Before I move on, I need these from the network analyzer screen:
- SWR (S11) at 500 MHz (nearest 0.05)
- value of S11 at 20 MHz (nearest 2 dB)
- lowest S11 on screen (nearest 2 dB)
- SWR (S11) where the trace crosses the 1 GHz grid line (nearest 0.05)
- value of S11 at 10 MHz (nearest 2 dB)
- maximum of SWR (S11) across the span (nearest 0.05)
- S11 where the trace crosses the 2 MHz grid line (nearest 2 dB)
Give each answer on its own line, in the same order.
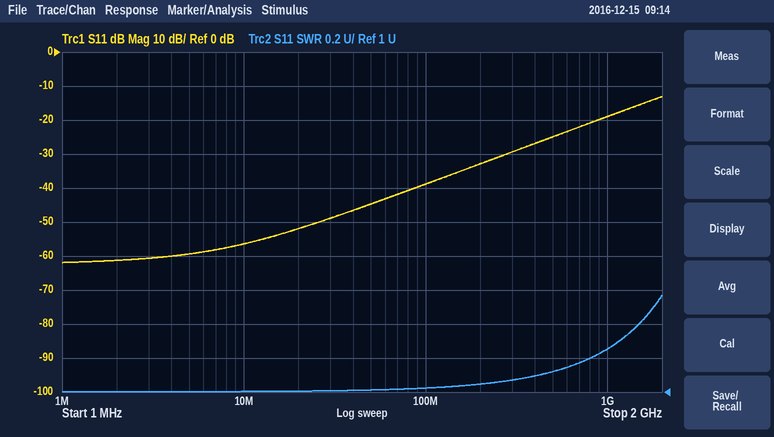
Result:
1.10
-52 dB
-62 dB
1.25
-56 dB
1.55
-62 dB
